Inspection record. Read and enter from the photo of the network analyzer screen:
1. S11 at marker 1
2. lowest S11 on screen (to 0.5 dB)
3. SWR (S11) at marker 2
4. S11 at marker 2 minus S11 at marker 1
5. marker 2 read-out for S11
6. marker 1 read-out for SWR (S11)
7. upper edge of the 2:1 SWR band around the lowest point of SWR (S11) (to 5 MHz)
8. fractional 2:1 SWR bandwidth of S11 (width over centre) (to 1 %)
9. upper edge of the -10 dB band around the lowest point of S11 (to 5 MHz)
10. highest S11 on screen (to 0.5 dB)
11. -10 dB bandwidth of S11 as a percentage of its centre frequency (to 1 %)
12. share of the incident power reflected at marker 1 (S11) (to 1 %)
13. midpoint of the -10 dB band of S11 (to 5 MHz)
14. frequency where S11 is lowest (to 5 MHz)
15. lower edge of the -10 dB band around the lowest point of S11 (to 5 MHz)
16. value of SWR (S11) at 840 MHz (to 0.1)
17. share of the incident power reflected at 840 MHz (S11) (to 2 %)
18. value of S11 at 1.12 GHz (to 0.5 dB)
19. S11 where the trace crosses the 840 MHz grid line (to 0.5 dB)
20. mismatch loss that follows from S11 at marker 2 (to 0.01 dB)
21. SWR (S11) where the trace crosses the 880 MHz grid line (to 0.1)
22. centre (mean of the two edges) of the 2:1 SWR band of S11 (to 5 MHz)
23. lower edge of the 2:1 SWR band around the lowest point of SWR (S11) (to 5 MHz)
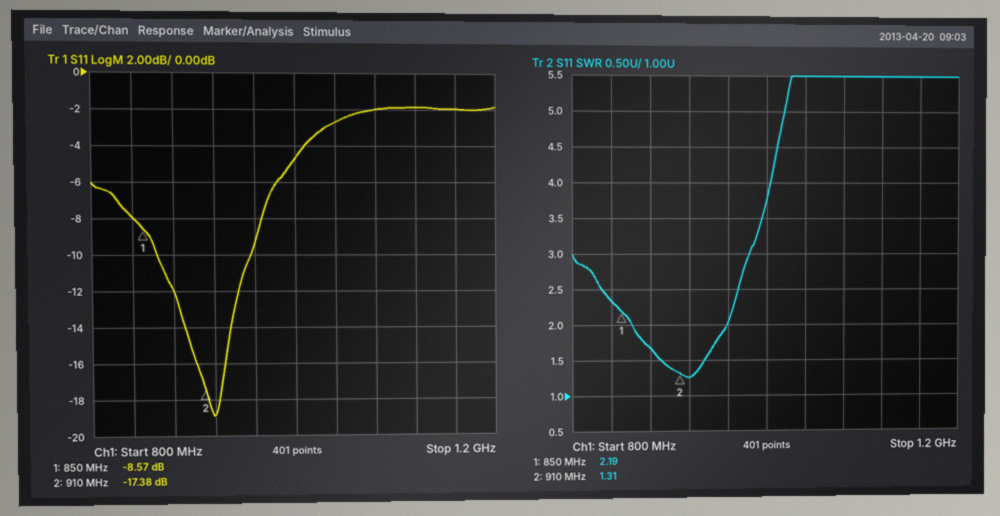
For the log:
-8.57 dB
-19.0 dB
1.31
-8.81 dB
-17.38 dB
2.19
960 MHz
11 %
955 MHz
-2.0 dB
10 %
14 %
910 MHz
920 MHz
865 MHz
2.3
16 %
-2.0 dB
-8.0 dB
0.08 dB
1.7
910 MHz
860 MHz
